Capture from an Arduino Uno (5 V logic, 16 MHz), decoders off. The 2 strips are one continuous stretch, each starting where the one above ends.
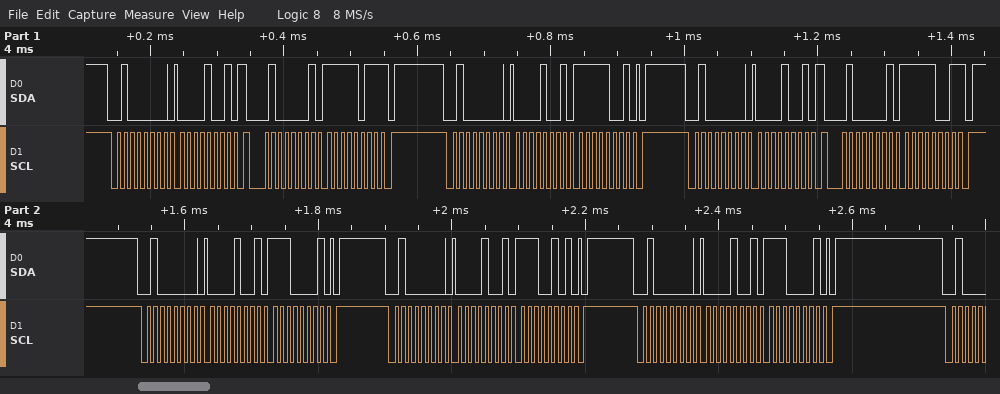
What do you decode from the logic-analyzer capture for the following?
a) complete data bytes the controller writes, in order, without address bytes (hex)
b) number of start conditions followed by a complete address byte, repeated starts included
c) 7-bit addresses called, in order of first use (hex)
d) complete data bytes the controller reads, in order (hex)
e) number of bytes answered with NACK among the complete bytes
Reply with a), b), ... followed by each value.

a) 09 09 F9 09 09 E1 09 E5 09 E1
b) 8
c) 0x20
d) FB F9
e) 2
